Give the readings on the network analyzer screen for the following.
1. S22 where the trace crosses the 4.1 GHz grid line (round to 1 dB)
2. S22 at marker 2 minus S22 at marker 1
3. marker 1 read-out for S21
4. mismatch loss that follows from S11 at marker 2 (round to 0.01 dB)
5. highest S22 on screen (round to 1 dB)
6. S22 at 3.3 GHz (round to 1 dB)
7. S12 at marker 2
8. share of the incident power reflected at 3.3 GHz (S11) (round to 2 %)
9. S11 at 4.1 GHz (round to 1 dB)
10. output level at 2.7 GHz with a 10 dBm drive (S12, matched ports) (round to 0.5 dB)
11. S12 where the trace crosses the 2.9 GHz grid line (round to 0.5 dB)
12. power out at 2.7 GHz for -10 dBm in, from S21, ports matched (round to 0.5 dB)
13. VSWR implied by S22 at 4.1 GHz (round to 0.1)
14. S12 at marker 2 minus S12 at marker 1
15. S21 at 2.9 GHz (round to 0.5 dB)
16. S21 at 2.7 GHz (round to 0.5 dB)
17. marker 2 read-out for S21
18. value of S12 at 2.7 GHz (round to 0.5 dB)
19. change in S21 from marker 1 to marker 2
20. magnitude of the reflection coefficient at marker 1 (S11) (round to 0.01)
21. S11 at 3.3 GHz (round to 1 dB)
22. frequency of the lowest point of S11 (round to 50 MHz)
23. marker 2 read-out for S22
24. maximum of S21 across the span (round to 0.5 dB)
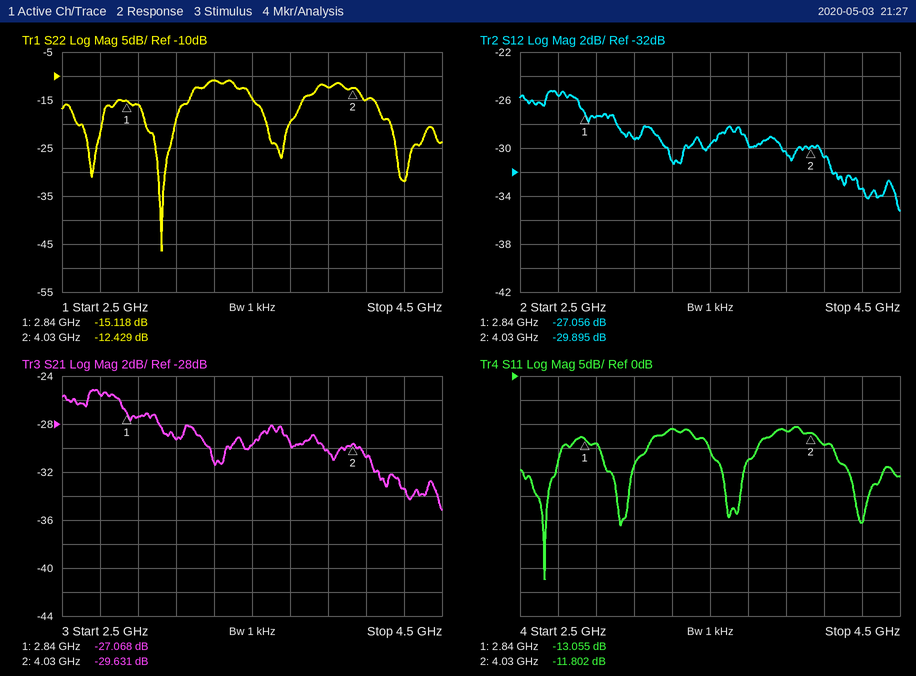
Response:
-15 dB
2.689 dB
-27.068 dB
0.30 dB
-11 dB
-11 dB
-29.895 dB
8 %
-14 dB
-15.5 dBm
-27.5 dB
-35.5 dBm
1.4
-2.839 dB
-27.5 dB
-25.5 dB
-29.631 dB
-25.5 dB
-2.563 dB
0.22
-11 dB
2.65 GHz
-12.429 dB
-25.0 dB
